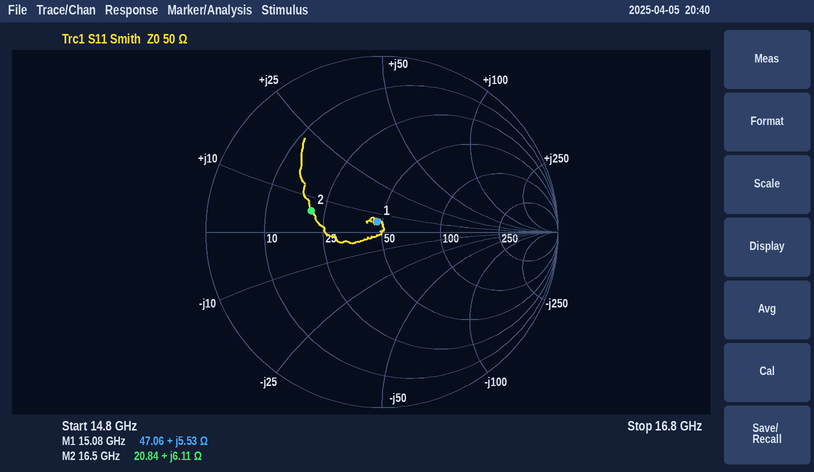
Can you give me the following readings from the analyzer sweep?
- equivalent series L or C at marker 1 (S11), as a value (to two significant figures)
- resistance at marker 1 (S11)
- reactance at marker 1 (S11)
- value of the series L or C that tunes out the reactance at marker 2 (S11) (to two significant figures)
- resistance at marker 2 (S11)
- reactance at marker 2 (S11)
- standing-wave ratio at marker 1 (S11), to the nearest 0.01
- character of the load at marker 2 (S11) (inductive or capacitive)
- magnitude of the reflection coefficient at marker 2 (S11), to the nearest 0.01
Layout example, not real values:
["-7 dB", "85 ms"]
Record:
["58 pH", "47.06 Ω", "+5.53 Ω", "1.6 pF", "20.84 Ω", "+6.11 Ω", "1.14", "inductive", "0.42"]
